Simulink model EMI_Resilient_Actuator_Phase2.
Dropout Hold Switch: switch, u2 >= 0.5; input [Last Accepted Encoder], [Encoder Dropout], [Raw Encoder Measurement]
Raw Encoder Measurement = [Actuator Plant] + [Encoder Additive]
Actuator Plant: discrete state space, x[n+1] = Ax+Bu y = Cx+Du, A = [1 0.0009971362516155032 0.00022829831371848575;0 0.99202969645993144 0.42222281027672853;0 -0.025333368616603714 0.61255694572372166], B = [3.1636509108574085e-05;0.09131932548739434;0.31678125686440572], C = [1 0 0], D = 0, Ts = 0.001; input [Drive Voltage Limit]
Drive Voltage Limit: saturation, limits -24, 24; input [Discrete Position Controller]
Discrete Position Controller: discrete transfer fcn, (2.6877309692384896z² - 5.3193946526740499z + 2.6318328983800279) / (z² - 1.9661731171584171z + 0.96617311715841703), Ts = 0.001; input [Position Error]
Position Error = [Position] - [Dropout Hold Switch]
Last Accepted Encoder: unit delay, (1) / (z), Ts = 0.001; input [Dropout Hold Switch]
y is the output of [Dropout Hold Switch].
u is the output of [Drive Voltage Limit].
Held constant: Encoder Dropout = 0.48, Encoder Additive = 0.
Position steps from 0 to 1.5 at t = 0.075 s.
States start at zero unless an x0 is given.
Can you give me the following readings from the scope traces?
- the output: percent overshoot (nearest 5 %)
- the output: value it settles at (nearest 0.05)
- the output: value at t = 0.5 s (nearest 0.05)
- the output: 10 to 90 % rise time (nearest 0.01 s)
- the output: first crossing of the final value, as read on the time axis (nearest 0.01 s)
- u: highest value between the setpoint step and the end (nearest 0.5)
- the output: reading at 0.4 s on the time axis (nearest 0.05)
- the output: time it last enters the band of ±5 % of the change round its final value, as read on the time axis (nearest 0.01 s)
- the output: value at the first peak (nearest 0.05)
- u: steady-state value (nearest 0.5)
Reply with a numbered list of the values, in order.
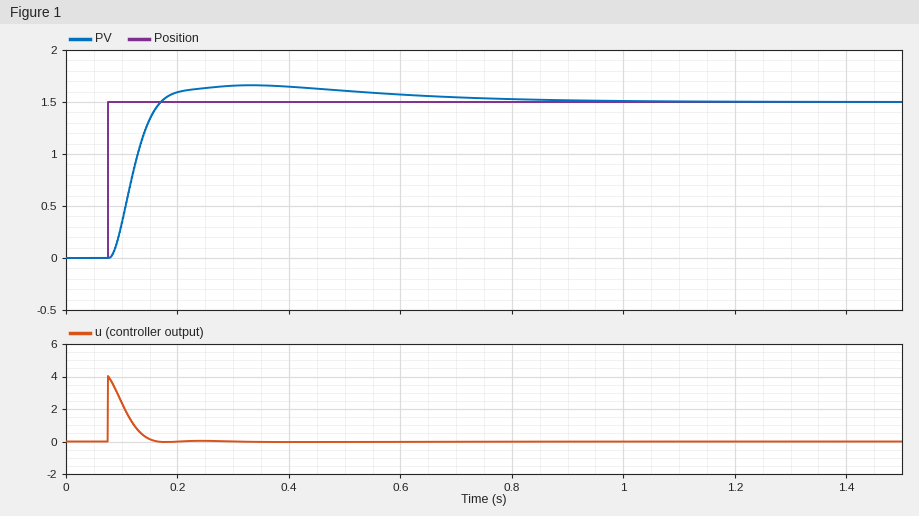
1. 10 %
2. 1.50
3. 1.60
4. 0.06 s
5. 0.17 s
6. 4.0
7. 1.65
8. 0.59 s
9. 1.65
10. 0.0
